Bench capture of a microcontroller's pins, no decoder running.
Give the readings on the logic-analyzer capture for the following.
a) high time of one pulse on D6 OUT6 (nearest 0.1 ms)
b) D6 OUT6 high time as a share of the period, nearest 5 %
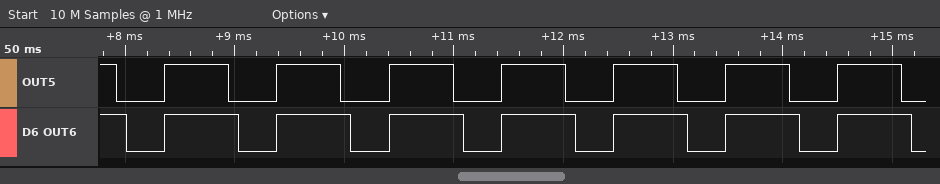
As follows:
0.7 ms
65 %
